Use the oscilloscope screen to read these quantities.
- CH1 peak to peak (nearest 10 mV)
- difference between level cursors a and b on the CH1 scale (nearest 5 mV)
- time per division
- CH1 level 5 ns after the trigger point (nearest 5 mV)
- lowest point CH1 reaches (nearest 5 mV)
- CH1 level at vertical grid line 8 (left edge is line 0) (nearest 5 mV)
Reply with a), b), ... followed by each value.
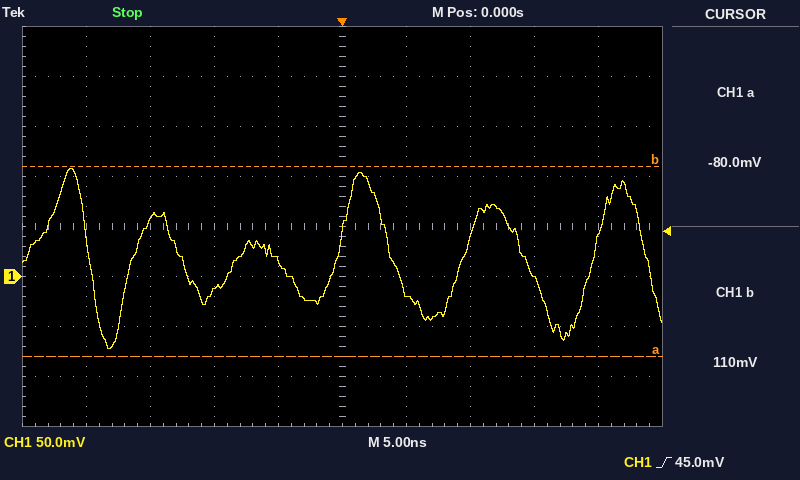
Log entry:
a) 180 mV
b) 190 mV
c) 5 ns
d) -15 mV
e) -70 mV
f) 0 mV
